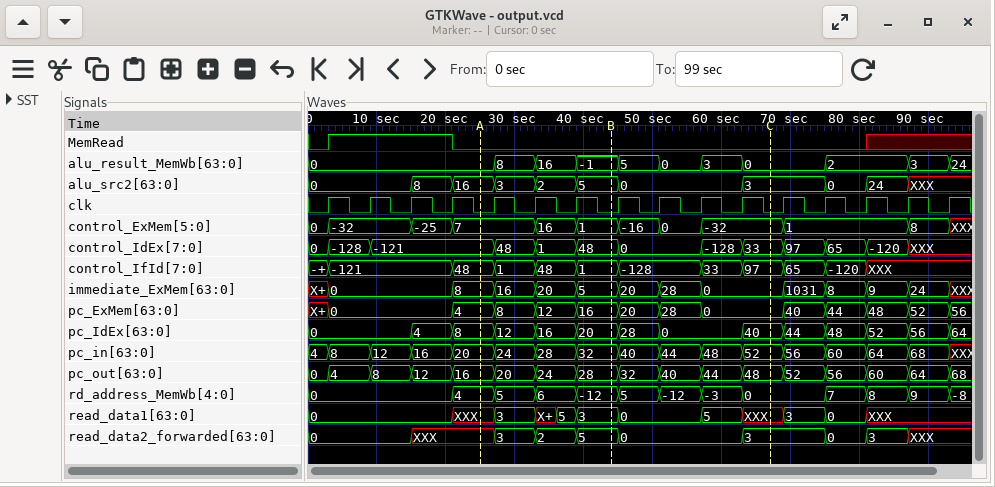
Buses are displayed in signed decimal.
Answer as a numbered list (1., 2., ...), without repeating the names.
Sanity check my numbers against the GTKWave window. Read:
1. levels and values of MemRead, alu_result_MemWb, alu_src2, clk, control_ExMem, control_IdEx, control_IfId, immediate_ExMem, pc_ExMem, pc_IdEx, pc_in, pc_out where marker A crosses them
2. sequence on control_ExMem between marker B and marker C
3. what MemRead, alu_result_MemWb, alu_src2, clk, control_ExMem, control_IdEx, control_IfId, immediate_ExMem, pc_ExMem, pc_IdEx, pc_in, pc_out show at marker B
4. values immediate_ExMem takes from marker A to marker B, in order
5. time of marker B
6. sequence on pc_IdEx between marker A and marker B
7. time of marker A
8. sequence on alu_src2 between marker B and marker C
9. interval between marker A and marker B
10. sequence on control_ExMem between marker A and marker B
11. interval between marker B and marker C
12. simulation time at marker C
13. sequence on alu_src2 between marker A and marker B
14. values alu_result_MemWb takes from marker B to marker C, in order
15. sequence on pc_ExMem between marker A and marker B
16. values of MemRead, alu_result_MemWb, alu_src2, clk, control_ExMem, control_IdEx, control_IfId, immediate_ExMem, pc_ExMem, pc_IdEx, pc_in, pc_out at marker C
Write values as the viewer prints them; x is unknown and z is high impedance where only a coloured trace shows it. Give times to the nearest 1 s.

1. MemRead=0, alu_result_MemWb=0, alu_src2=16, clk=0, control_ExMem=7, control_IdEx=-121, control_IfId=48, immediate_ExMem=8, pc_ExMem=4, pc_IdEx=8, pc_in=20, pc_out=16
2. 1, -16, 0, -32
3. MemRead=0, alu_result_MemWb=-1, alu_src2=5, clk=0, control_ExMem=1, control_IdEx=48, control_IfId=1, immediate_ExMem=5, pc_ExMem=16, pc_IdEx=20, pc_in=32, pc_out=28
4. 8, 16, 20, 5
5. 44 s
6. 8, 12, 16, 20
7. 25 s
8. 5, 0, 3
9. 19 s
10. 7, 16, 1
11. 23 s
12. 67 s
13. 16, 3, 2, 5
14. -1, 5, 0, 3, 0
15. 4, 8, 12, 16
16. MemRead=0, alu_result_MemWb=0, alu_src2=3, clk=0, control_ExMem=-32, control_IdEx=33, control_IfId=97, immediate_ExMem=0, pc_ExMem=0, pc_IdEx=40, pc_in=52, pc_out=48
